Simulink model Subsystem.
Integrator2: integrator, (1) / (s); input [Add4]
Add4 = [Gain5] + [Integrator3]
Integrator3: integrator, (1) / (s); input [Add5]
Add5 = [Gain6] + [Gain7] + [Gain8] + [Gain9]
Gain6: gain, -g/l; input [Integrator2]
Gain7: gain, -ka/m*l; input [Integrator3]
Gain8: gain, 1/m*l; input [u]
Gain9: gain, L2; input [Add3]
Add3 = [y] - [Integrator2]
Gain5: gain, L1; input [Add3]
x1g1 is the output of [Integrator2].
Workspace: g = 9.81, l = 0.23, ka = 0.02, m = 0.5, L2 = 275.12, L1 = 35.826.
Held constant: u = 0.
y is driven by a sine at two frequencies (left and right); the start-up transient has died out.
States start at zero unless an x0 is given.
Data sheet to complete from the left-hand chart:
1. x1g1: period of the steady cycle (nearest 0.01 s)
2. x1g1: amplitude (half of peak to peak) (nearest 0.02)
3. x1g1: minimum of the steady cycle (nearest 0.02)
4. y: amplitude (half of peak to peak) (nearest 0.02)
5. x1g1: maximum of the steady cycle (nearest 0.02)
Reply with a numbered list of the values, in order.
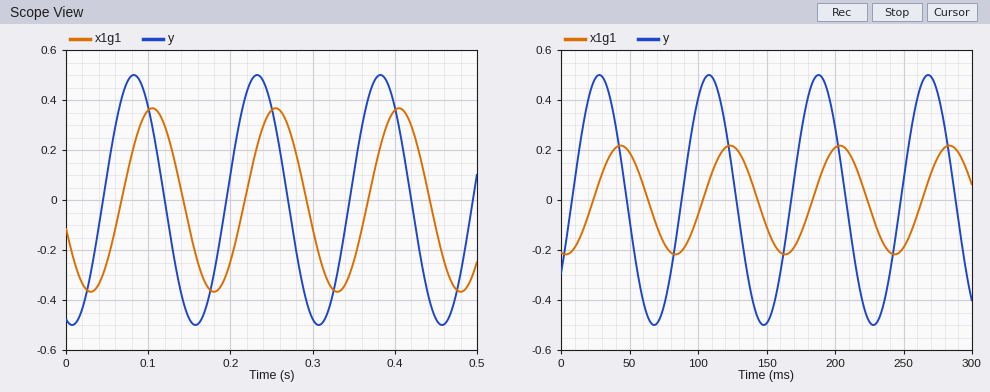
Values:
1. 0.15 s
2. 0.36
3. -0.36
4. 0.50
5. 0.36
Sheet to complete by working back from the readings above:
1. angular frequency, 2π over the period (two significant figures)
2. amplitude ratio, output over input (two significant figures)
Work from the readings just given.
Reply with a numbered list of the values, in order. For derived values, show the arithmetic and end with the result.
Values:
1. 2π / 0.15 = 42 rad/s
2. 0.36 / 0.5 = 0.72
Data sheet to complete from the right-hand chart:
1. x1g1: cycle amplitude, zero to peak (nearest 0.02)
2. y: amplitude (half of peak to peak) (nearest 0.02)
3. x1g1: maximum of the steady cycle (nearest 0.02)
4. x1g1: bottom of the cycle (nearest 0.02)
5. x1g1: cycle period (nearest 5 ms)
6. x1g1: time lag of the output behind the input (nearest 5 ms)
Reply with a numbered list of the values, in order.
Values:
1. 0.22
2. 0.50
3. 0.22
4. -0.22
5. 80 ms
6. 15 ms
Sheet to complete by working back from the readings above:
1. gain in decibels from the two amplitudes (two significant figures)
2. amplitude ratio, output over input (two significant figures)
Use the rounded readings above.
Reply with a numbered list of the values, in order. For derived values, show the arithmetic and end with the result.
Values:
1. 20 log10(0.22 / 0.5) = -7.1 dB
2. 0.22 / 0.5 = 0.44
